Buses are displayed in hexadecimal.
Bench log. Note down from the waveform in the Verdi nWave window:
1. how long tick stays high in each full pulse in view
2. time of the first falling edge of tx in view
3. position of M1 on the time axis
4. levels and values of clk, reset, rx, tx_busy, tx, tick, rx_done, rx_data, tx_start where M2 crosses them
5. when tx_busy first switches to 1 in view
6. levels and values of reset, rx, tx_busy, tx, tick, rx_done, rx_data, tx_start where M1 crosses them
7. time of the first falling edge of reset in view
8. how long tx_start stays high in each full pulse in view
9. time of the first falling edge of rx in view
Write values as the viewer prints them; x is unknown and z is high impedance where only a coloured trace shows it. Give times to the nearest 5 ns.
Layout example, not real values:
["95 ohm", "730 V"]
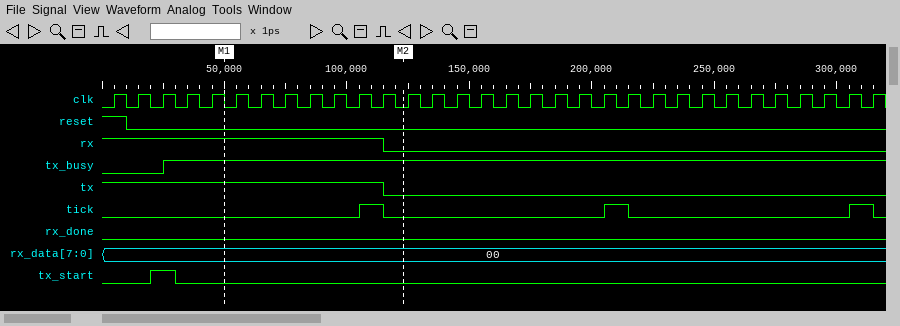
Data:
["10 ns, 10 ns, 10 ns", "115 ns", "50 ns", "clk=0, reset=0, rx=0, tx_busy=1, tx=0, tick=0, rx_done=0, rx_data=00, tx_start=0", "25 ns", "reset=0, rx=1, tx_busy=1, tx=1, tick=0, rx_done=0, rx_data=00, tx_start=0", "10 ns", "10 ns", "115 ns"]
